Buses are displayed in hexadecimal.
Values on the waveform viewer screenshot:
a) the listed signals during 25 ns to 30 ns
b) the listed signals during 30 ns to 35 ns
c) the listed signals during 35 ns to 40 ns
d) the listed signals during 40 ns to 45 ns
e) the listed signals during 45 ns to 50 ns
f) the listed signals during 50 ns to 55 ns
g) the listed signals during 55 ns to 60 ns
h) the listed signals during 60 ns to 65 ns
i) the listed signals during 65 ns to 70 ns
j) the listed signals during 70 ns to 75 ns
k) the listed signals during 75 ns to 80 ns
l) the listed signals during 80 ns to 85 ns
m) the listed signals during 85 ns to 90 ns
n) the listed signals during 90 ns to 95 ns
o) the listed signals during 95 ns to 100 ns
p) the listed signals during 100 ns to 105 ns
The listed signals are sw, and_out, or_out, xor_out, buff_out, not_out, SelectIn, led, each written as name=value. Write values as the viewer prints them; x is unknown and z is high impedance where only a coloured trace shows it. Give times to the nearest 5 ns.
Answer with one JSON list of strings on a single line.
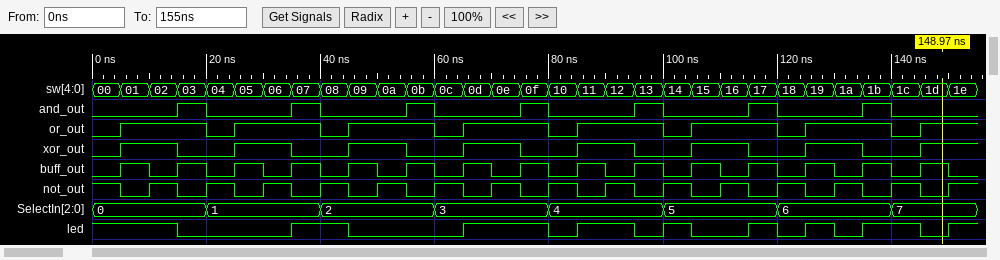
["sw=05, and_out=0, or_out=1, xor_out=1, buff_out=1, not_out=0, SelectIn=1, led=0", "sw=06, and_out=0, or_out=1, xor_out=1, buff_out=0, not_out=1, SelectIn=1, led=0", "sw=07, and_out=1, or_out=1, xor_out=0, buff_out=1, not_out=0, SelectIn=1, led=1", "sw=08, and_out=0, or_out=0, xor_out=0, buff_out=0, not_out=1, SelectIn=2, led=1", "sw=09, and_out=0, or_out=1, xor_out=1, buff_out=1, not_out=0, SelectIn=2, led=0", "sw=0a, and_out=0, or_out=1, xor_out=1, buff_out=0, not_out=1, SelectIn=2, led=0", "sw=0b, and_out=1, or_out=1, xor_out=0, buff_out=1, not_out=0, SelectIn=2, led=0", "sw=0c, and_out=0, or_out=0, xor_out=0, buff_out=0, not_out=1, SelectIn=3, led=0", "sw=0d, and_out=0, or_out=1, xor_out=1, buff_out=1, not_out=0, SelectIn=3, led=1", "sw=0e, and_out=0, or_out=1, xor_out=1, buff_out=0, not_out=1, SelectIn=3, led=1", "sw=0f, and_out=1, or_out=1, xor_out=0, buff_out=1, not_out=0, SelectIn=3, led=1", "sw=10, and_out=0, or_out=0, xor_out=0, buff_out=0, not_out=1, SelectIn=4, led=0", "sw=11, and_out=0, or_out=1, xor_out=1, buff_out=1, not_out=0, SelectIn=4, led=1", "sw=12, and_out=0, or_out=1, xor_out=1, buff_out=0, not_out=1, SelectIn=4, led=1", "sw=13, and_out=1, or_out=1, xor_out=0, buff_out=1, not_out=0, SelectIn=4, led=0", "sw=14, and_out=0, or_out=0, xor_out=0, buff_out=0, not_out=1, SelectIn=5, led=1"]
